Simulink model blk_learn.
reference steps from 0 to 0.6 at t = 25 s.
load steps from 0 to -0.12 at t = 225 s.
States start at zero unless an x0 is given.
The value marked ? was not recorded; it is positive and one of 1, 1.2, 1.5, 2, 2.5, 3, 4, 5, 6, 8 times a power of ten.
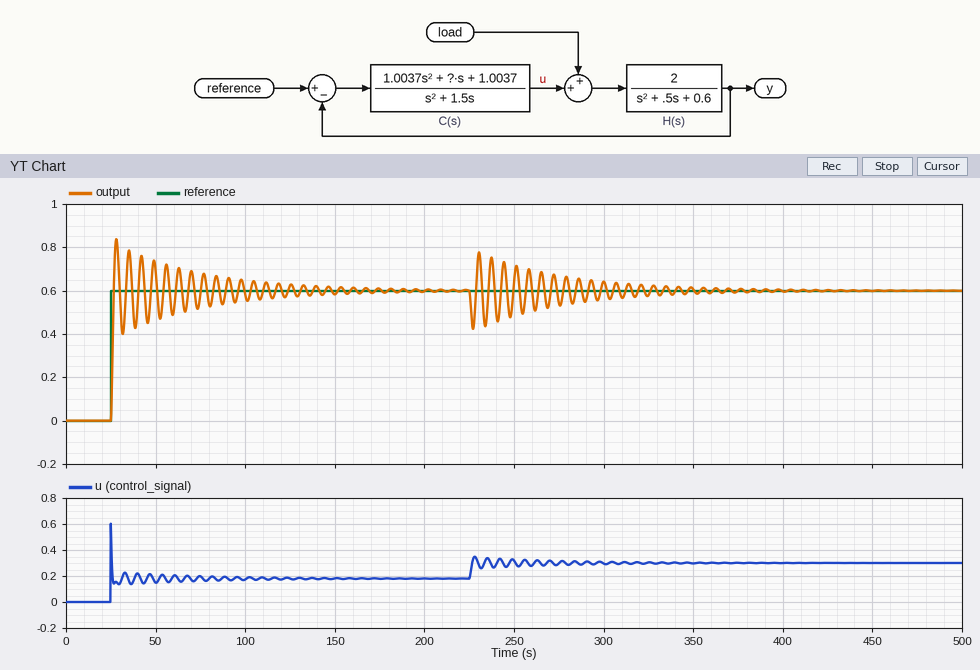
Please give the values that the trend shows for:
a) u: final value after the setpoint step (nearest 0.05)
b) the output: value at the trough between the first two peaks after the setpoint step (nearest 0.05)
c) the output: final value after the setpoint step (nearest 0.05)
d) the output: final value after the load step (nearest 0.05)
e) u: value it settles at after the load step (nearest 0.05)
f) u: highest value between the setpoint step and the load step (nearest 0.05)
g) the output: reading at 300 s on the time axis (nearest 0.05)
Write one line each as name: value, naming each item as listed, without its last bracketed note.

u: final value after the setpoint step: 0.20
the output: value at the trough between the first two peaks after the setpoint step: 0.40
the output: final value after the setpoint step: 0.60
the output: final value after the load step: 0.60
u: value it settles at after the load step: 0.30
u: highest value between the setpoint step and the load step: 0.60
the output: reading at 300 s on the time axis: 0.65
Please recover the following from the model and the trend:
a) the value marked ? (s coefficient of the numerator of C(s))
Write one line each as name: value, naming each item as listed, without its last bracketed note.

the value marked ? (s coefficient of the numerator of C(s)): 0.4
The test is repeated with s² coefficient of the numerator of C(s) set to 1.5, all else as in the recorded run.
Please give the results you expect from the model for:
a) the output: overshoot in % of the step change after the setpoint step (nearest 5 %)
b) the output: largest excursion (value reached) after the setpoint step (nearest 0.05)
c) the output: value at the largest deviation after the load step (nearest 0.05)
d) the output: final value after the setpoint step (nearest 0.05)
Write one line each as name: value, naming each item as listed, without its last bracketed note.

the output: overshoot in % of the step change after the setpoint step: 15 %
the output: largest excursion (value reached) after the setpoint step: 0.70
the output: value at the largest deviation after the load step: 0.45
the output: final value after the setpoint step: 0.60
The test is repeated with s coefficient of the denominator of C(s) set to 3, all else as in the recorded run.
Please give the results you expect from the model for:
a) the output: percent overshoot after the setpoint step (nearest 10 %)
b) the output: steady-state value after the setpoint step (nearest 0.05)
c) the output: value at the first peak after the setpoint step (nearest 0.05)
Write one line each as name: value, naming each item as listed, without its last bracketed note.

the output: percent overshoot after the setpoint step: 30 %
the output: steady-state value after the setpoint step: 0.60
the output: value at the first peak after the setpoint step: 0.75
